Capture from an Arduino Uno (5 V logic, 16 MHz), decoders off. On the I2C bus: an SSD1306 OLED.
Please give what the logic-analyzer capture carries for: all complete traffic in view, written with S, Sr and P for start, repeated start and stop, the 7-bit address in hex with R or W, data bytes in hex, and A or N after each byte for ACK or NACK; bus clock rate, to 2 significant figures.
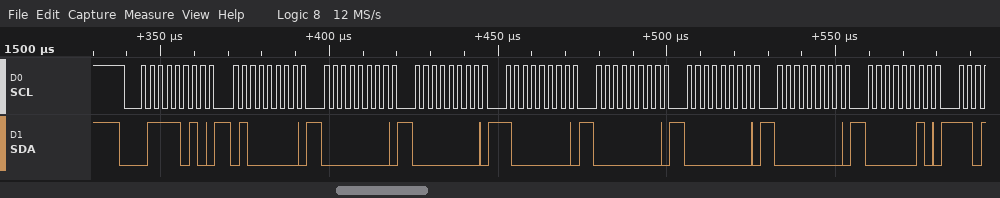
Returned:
S 3DW A 40 A 00 A 00 A 80 A 00 A 00 A 00 A 02 A
400 kHz
